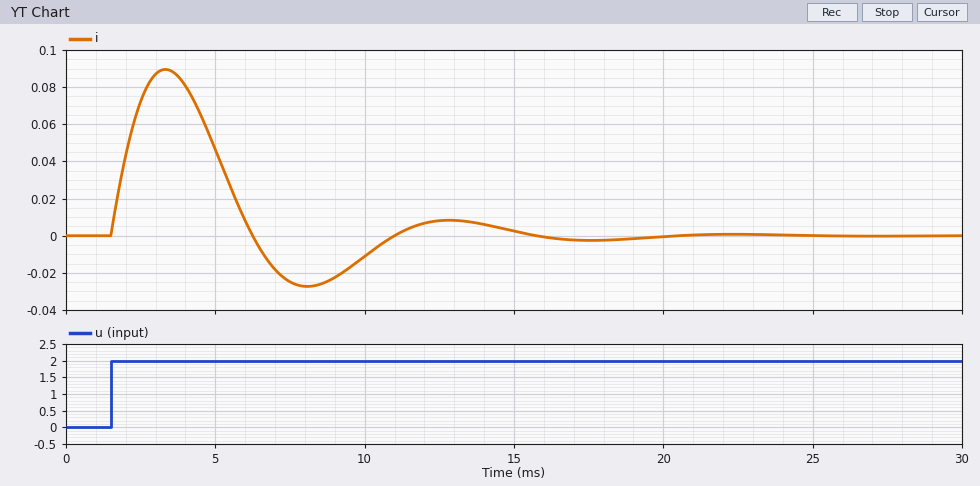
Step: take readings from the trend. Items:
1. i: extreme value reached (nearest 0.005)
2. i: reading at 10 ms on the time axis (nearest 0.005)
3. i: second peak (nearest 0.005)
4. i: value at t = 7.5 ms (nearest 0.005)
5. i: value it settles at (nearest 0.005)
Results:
0.090
-0.010
0.010
-0.025
0.000
